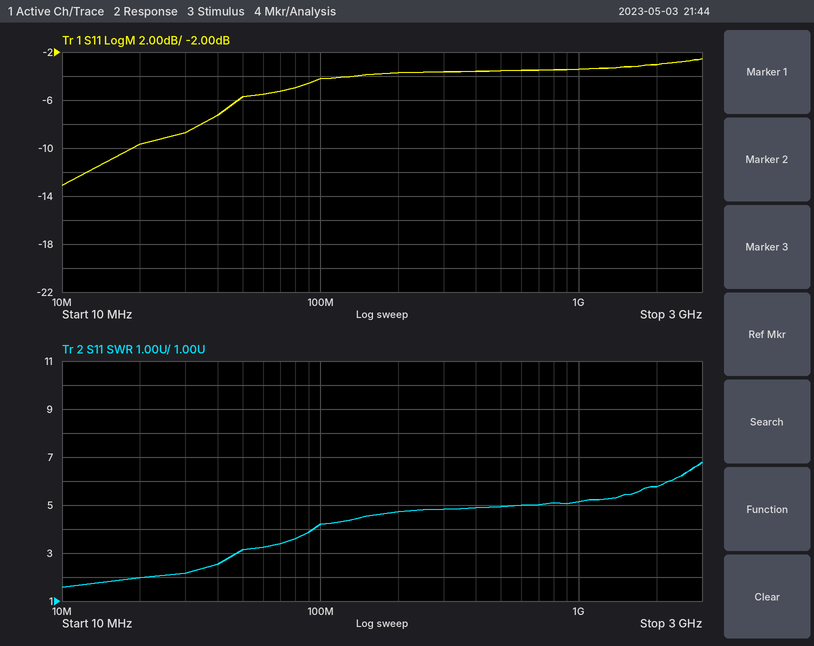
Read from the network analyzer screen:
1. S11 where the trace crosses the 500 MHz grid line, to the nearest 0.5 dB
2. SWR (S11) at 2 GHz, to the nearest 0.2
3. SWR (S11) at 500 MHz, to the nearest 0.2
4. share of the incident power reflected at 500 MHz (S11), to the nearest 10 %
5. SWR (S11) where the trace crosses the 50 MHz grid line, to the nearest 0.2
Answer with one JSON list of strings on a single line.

["-3.5 dB", "5.8", "5.0", "40 %", "3.2"]
